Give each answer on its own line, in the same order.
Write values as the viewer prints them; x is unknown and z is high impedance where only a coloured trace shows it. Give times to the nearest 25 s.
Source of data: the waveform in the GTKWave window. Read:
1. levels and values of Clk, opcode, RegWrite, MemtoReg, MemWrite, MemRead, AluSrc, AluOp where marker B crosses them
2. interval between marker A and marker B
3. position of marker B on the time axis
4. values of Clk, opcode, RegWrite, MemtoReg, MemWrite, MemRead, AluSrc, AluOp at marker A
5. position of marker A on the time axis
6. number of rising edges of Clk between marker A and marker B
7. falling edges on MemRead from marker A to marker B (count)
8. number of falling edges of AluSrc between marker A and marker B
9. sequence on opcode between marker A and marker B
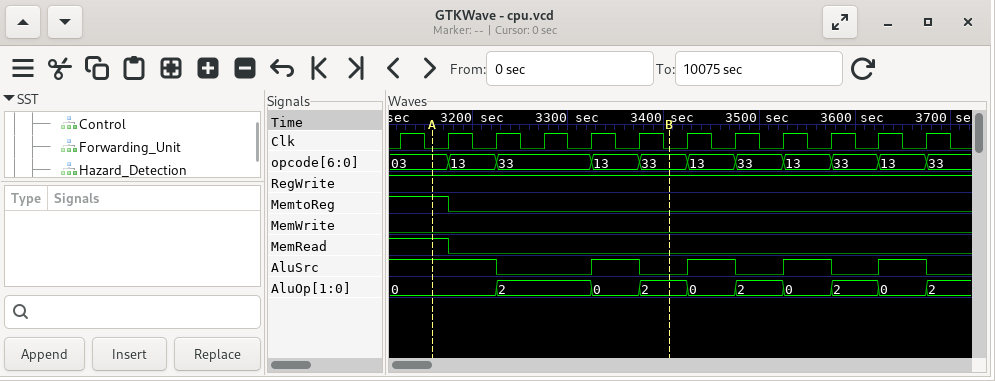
Clk=0, opcode=33, RegWrite=1, MemtoReg=0, MemWrite=0, MemRead=0, AluSrc=0, AluOp=2
250 s
3400 s
Clk=0, opcode=03, RegWrite=1, MemtoReg=1, MemWrite=0, MemRead=1, AluSrc=1, AluOp=0
3150 s
5
1
2
03, 13, 33, 13, 33
